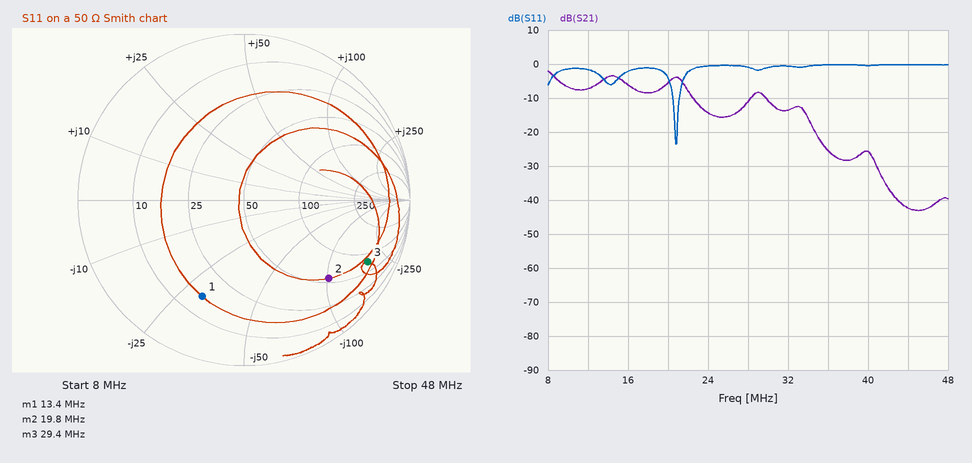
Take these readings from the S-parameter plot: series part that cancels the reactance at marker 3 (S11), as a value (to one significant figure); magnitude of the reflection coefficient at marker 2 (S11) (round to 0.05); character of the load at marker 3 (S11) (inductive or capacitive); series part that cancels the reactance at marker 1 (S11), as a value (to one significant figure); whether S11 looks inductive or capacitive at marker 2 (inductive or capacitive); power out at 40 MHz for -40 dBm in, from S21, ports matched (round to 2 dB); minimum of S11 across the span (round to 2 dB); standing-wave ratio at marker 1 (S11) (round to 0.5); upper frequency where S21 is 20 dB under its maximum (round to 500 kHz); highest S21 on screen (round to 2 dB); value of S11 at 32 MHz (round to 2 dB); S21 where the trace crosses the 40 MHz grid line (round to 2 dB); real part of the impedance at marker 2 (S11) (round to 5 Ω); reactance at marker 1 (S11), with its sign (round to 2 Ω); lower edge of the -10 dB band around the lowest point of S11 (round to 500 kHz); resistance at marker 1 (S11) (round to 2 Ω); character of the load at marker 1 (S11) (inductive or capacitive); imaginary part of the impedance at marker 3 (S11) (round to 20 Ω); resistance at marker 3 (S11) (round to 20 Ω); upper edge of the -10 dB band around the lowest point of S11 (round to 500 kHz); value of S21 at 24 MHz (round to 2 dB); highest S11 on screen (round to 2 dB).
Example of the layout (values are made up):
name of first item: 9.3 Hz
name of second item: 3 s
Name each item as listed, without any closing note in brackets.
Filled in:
series part that cancels the reactance at marker 3 (S11), as a value: 1.0 µH
magnitude of the reflection coefficient at marker 2 (S11): 0.70
character of the load at marker 3 (S11): capacitive
series part that cancels the reactance at marker 1 (S11), as a value: 400 nH
whether S11 looks inductive or capacitive at marker 2: capacitive
power out at 40 MHz for -40 dBm in, from S21, ports matched: -66 dBm
minimum of S11 across the span: -24 dB
standing-wave ratio at marker 1 (S11): 4.5
upper frequency where S21 is 20 dB under its maximum: 35.0 MHz
highest S21 on screen: -2 dB
value of S11 at 32 MHz: 0 dB
S21 where the trace crosses the 40 MHz grid line: -26 dB
real part of the impedance at marker 2 (S11): 55 Ω
reactance at marker 1 (S11), with its sign: -30 Ω
lower edge of the -10 dB band around the lowest point of S11: 20.5 MHz
resistance at marker 1 (S11): 16 Ω
character of the load at marker 1 (S11): capacitive
imaginary part of the impedance at marker 3 (S11): -180 Ω
resistance at marker 3 (S11): 80 Ω
upper edge of the -10 dB band around the lowest point of S11: 21.0 MHz
value of S21 at 24 MHz: -14 dB
highest S11 on screen: 0 dB
